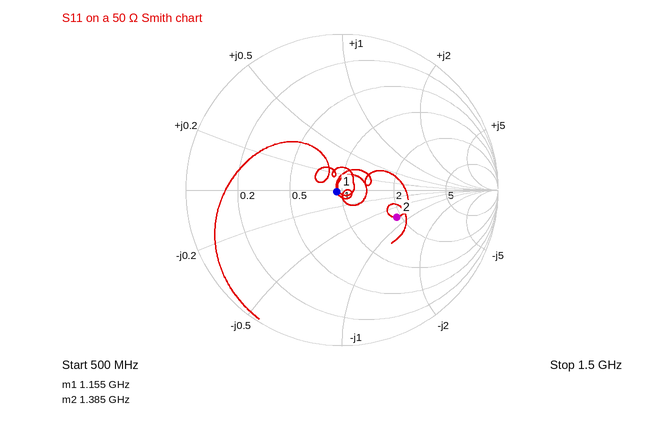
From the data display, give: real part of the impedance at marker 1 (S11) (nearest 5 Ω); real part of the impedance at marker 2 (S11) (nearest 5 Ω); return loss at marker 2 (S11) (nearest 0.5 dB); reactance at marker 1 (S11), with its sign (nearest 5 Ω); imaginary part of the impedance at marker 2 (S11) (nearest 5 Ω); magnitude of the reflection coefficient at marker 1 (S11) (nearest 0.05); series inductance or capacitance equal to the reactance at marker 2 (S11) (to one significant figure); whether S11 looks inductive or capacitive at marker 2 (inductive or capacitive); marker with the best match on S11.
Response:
45 Ω
95 Ω
8.0 dB
0 Ω
-40 Ω
0.05
3 pF
capacitive
marker 1
